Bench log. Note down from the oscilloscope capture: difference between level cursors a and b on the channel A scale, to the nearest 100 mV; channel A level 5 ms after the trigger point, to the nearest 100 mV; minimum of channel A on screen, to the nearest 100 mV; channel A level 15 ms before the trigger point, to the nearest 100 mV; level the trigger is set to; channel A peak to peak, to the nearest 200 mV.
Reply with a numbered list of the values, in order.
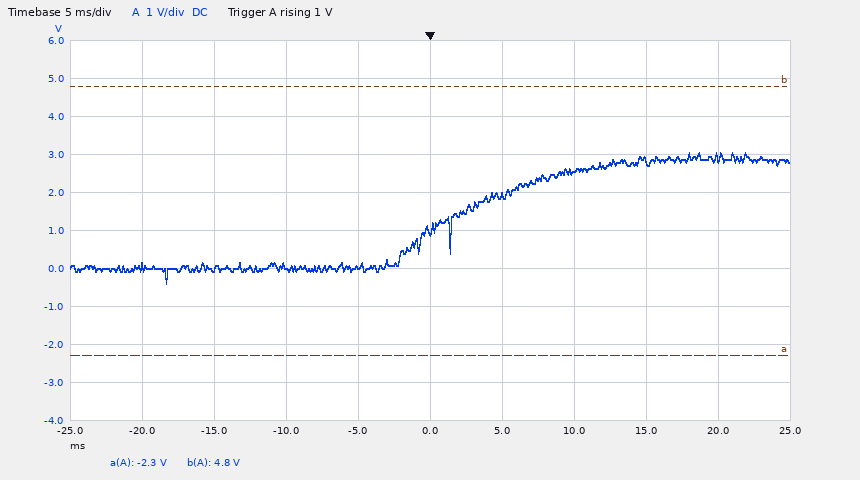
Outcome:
1. 7.1 V
2. 1.9 V
3. -400 mV
4. 0.0 V
5. 1 V
6. 3.4 V
